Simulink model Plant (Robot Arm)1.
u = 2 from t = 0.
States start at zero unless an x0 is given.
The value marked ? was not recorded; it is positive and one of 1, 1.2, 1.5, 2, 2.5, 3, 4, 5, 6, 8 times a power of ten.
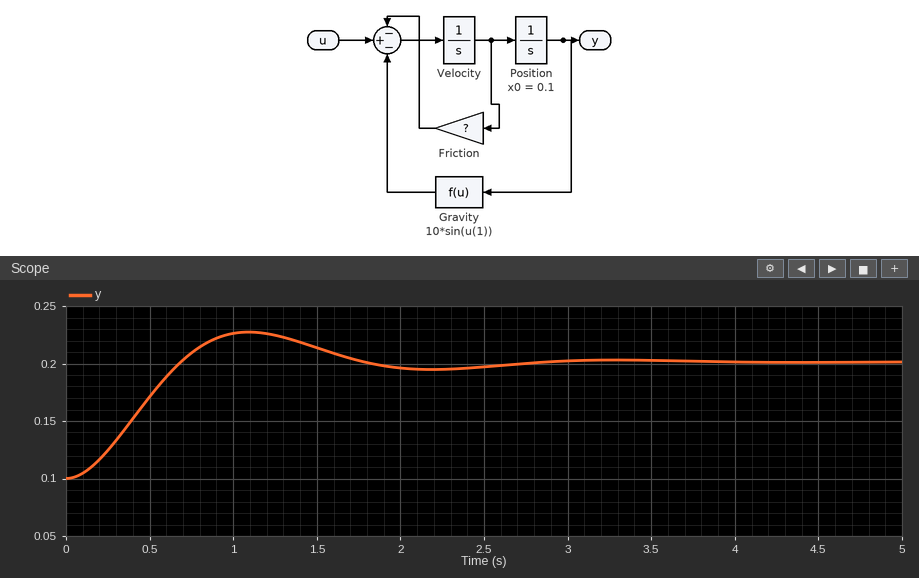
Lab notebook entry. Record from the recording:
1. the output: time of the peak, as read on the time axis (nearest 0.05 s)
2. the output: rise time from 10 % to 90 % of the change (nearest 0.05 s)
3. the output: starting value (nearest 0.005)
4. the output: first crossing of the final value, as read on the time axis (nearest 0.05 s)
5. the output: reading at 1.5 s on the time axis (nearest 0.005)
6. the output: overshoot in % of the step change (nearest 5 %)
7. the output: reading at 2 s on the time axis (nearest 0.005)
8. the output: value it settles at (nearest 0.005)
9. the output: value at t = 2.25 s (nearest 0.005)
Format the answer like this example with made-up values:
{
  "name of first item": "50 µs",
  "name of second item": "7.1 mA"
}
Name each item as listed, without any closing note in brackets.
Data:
{
  "the output: time of the peak, as read on the time axis": "1.10 s",
  "the output: rise time from 10 % to 90 % of the change": "0.45 s",
  "the output: starting value": "0.100",
  "the output: first crossing of the final value, as read on the time axis": "0.70 s",
  "the output: reading at 1.5 s on the time axis": "0.215",
  "the output: overshoot in % of the step change": "25 %",
  "the output: reading at 2 s on the time axis": "0.195",
  "the output: value it settles at": "0.200",
  "the output: value at t = 2.25 s": "0.195"
}
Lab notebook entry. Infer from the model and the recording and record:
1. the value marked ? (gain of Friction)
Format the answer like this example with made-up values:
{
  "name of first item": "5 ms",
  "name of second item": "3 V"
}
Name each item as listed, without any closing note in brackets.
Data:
{
  "the value marked ?": "2.5"
}
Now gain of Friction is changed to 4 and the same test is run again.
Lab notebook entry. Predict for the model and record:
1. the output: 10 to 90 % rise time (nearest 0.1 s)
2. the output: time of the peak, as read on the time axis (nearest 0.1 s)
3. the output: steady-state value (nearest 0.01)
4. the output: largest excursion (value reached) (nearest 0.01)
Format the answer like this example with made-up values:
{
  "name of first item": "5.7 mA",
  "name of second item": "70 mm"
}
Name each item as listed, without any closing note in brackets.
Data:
{
  "the output: 10 to 90 % rise time": "0.6 s",
  "the output: time of the peak, as read on the time axis": "1.3 s",
  "the output: steady-state value": "0.20",
  "the output: largest excursion (value reached)": "0.21"
}
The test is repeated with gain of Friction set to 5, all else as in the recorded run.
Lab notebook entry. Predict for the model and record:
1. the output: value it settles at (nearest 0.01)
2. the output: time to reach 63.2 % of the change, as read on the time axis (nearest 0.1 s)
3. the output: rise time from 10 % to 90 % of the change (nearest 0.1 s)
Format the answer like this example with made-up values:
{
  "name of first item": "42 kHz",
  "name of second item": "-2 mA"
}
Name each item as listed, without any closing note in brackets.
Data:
{
  "the output: value it settles at": "0.20",
  "the output: time to reach 63.2 % of the change, as read on the time axis": "0.6 s",
  "the output: rise time from 10 % to 90 % of the change": "0.8 s"
}
